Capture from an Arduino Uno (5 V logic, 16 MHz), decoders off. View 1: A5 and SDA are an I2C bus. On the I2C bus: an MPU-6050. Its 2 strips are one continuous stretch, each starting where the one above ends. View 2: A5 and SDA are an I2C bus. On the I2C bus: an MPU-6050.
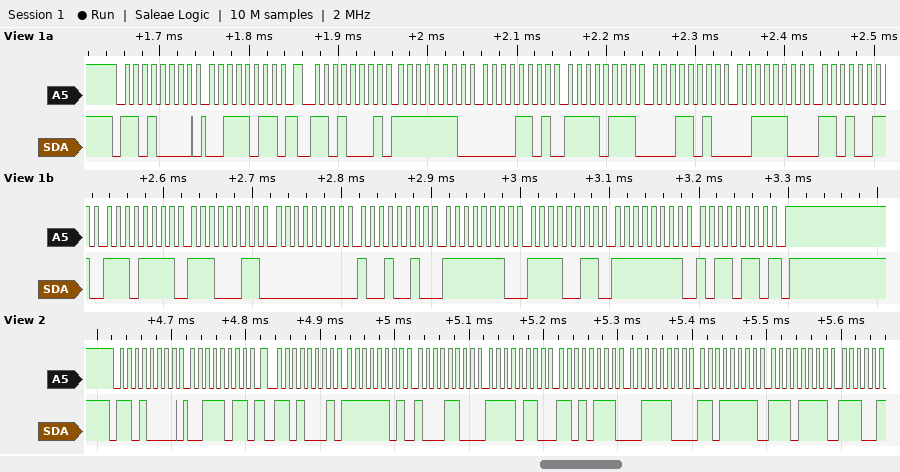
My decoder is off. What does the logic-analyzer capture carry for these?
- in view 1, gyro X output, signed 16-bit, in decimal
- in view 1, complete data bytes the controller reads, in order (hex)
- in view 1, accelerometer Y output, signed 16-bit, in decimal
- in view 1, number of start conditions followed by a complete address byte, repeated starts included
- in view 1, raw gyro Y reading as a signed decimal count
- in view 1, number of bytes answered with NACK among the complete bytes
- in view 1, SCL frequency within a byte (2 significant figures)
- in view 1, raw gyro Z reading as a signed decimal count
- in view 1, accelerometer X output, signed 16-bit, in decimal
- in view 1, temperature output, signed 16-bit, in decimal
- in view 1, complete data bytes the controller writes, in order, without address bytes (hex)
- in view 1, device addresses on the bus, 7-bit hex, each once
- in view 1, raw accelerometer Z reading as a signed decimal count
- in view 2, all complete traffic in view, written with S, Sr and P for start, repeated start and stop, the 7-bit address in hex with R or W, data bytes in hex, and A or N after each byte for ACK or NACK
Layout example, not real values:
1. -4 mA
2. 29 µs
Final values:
1. 146
2. FE 0D F7 1A 3C D3 EF E3 00 92 FE F3 FF B6
3. -2278
4. 2
5. -269
6. 1
7. 100 kHz
8. -74
9. -499
10. -4125
11. 3B
12. 0x68
13. 15571
14. S 68W A 3B A Sr 68R A FD A 8C A F6 A D7 A 3C A DF A EF A
